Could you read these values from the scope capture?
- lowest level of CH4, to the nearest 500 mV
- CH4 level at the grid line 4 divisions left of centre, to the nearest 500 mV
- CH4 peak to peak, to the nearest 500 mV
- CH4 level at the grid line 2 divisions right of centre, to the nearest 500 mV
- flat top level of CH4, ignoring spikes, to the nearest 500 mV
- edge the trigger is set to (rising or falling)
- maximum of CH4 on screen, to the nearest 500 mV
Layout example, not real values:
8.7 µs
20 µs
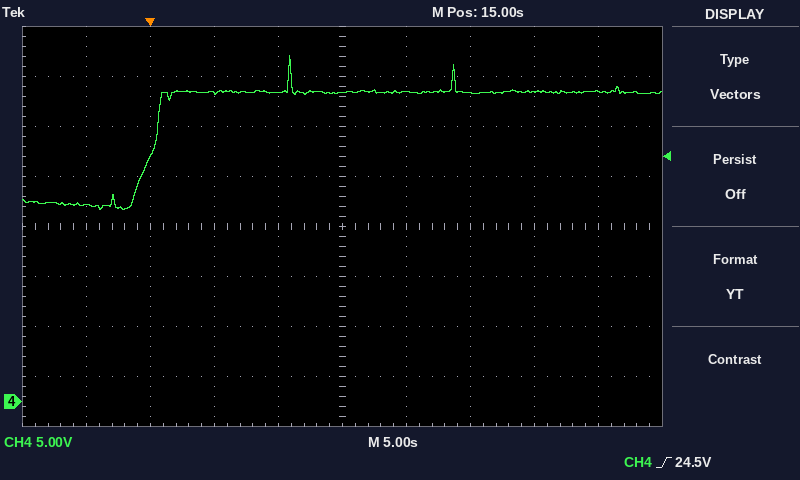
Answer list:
19.0 V
19.5 V
15.5 V
31.0 V
31.0 V
rising
34.5 V
